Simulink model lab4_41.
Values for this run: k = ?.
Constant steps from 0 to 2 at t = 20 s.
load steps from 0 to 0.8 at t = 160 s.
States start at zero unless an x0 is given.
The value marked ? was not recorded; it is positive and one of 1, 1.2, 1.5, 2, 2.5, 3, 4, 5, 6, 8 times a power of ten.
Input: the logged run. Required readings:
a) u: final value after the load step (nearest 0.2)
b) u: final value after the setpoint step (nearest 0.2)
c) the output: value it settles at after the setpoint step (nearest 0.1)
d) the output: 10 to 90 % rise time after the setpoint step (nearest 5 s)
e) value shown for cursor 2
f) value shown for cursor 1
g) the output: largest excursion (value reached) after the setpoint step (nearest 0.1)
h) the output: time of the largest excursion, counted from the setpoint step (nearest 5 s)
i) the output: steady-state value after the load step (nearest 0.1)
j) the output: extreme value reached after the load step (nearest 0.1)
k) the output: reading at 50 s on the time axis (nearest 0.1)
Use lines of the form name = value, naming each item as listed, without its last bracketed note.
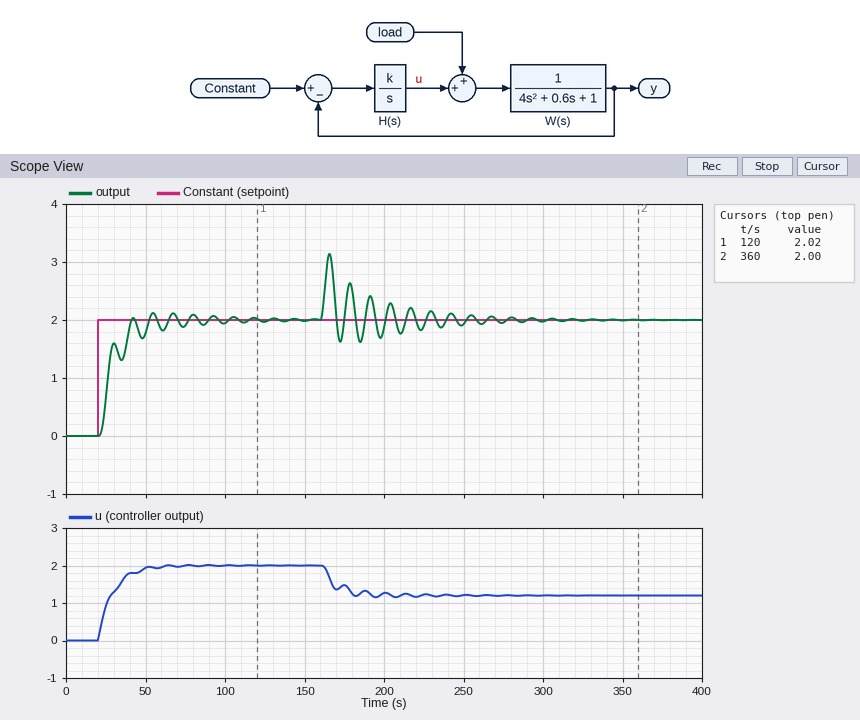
u: final value after the load step = 1.2
u: final value after the setpoint step = 2.0
the output: value it settles at after the setpoint step = 2.0
the output: 10 to 90 % rise time after the setpoint step = 15 s
value shown for cursor 2 = 2.00
value shown for cursor 1 = 2.02
the output: largest excursion (value reached) after the setpoint step = 2.1
the output: time of the largest excursion, counted from the setpoint step = 35 s
the output: steady-state value after the load step = 2.0
the output: extreme value reached after the load step = 3.1
the output: reading at 50 s on the time axis = 1.8
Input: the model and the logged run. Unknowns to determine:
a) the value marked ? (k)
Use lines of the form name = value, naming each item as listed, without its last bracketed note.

the value marked ? = 0.1
